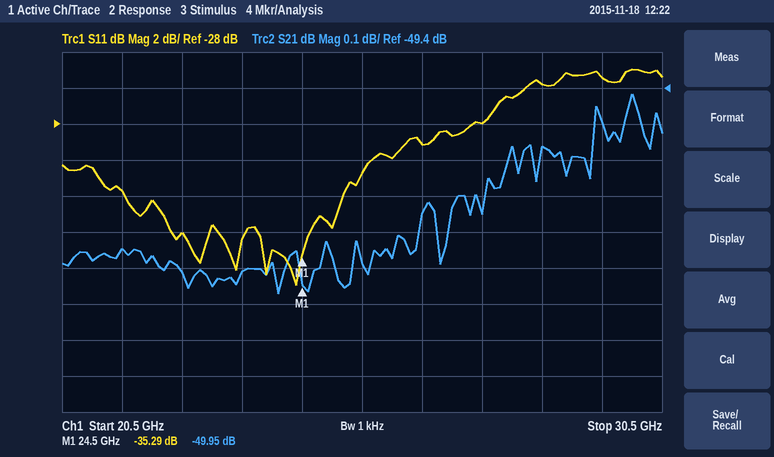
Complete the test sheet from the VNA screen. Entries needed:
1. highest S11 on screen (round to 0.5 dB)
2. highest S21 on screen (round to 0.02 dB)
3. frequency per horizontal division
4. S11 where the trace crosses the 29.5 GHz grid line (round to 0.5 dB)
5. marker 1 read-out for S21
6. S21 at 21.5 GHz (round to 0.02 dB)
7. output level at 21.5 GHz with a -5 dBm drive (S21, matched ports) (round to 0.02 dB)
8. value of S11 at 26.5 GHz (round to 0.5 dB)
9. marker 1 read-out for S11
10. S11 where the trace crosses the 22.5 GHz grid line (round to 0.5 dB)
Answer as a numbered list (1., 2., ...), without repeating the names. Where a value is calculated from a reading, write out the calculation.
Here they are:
1. -25.0 dB
2. -49.42 dB
3. 1 GHz
4. -25.5 dB
5. -49.95 dB
6. -49.84 dB
7. -5 dBm + (-49.84 dB) = -54.84 dBm
8. -29.0 dB
9. -35.29 dB
10. -34.0 dB
